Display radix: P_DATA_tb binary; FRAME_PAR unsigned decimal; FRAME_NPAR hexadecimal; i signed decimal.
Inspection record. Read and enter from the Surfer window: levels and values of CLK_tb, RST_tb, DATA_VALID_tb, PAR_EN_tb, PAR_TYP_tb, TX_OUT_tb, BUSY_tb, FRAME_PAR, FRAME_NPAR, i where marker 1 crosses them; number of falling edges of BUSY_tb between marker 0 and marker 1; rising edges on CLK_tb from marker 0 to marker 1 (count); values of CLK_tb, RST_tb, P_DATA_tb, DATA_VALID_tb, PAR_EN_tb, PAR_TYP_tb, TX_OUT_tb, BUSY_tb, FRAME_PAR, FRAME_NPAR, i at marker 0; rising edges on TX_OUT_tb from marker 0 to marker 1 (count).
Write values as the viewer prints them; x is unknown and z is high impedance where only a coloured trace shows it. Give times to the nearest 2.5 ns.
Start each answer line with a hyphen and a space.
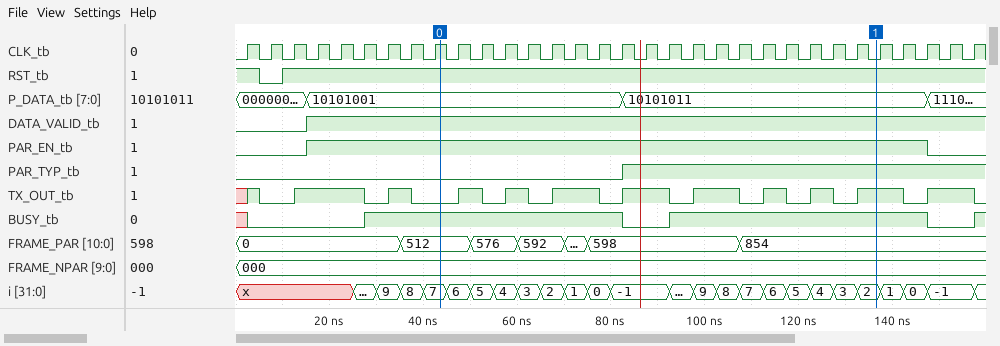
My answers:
- CLK_tb=0, RST_tb=1, DATA_VALID_tb=1, PAR_EN_tb=1, PAR_TYP_tb=1, TX_OUT_tb=1, BUSY_tb=1, FRAME_PAR=854, FRAME_NPAR=000, i=2
- 1
- 18
- CLK_tb=1, RST_tb=1, P_DATA_tb=10101001, DATA_VALID_tb=1, PAR_EN_tb=1, PAR_TYP_tb=0, TX_OUT_tb=0, BUSY_tb=1, FRAME_PAR=512, FRAME_NPAR=000, i=7
- 8
